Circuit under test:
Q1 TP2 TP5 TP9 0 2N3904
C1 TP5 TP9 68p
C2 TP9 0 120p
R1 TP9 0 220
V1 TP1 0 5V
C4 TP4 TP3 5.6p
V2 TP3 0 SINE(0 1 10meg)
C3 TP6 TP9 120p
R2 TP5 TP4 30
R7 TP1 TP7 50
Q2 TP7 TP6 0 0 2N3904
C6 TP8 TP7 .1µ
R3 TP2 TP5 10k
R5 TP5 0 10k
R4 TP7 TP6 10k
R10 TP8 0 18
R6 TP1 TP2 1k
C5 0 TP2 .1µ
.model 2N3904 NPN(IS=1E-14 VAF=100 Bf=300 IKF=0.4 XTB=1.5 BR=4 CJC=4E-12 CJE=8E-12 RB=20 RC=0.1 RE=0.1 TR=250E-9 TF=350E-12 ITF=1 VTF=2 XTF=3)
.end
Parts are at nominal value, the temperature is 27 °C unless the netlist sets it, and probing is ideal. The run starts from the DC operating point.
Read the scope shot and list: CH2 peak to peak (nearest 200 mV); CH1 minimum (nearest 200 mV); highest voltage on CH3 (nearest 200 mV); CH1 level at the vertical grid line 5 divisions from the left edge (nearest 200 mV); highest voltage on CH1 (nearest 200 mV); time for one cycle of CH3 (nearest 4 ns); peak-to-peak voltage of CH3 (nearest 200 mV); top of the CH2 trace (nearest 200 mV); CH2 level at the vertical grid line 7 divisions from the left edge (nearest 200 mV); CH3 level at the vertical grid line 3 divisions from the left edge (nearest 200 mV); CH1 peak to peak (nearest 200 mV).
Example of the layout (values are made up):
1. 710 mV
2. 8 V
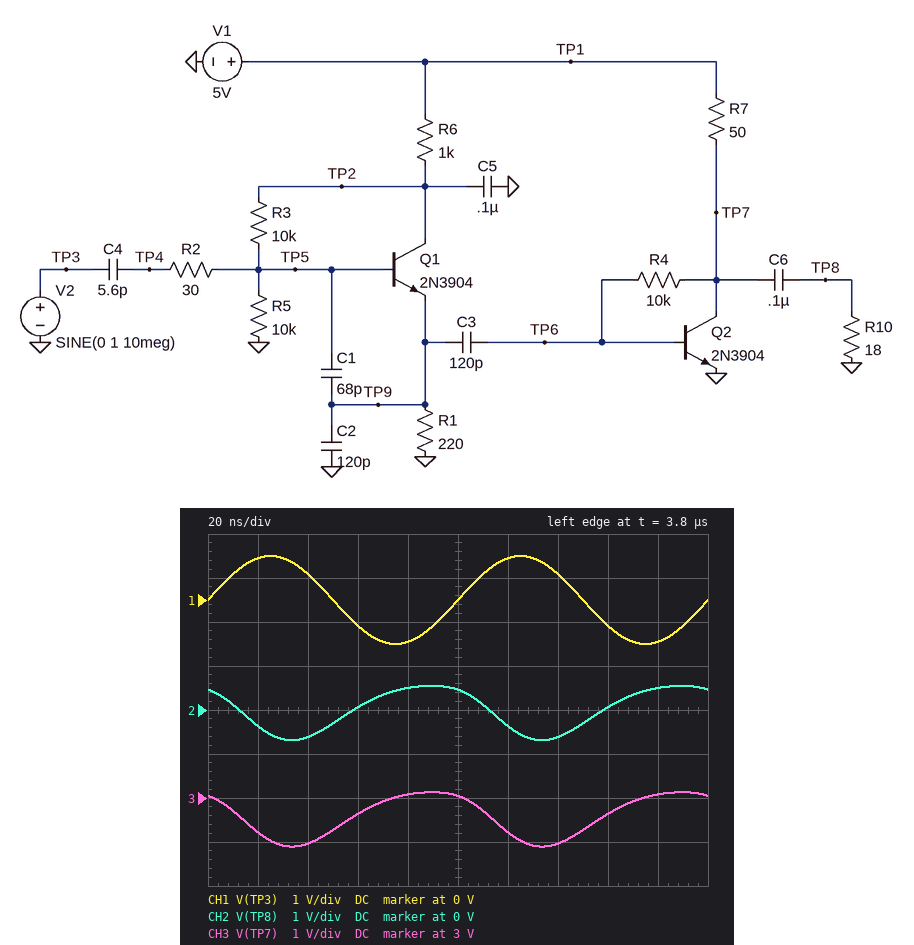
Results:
1. 1.2 V
2. -1.0 V
3. 3.2 V
4. 0 V
5. 1.0 V
6. 100 ns
7. 1.2 V
8. 600 mV
9. -600 mV
10. 2.6 V
11. 2.0 V
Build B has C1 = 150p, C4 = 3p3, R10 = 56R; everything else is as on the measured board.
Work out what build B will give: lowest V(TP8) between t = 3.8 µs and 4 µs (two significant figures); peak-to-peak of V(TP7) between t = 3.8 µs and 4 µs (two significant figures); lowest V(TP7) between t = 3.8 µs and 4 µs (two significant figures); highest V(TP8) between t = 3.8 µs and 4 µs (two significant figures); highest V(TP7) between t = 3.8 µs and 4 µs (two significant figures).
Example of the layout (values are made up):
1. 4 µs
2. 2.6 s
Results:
1. -570 mV
2. 1.1 V
3. 2.0 V
4. 520 mV
5. 3.1 V
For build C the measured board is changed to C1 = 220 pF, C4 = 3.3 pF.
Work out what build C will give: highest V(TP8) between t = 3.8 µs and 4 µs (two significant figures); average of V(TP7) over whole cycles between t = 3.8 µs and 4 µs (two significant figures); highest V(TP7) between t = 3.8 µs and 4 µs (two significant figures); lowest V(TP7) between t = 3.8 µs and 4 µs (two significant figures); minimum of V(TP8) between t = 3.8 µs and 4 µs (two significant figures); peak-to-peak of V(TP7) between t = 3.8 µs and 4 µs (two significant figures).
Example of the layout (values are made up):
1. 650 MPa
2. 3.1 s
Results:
1. 220 mV
2. 2.6 V
3. 2.8 V
4. 2.3 V
5. -240 mV
6. 450 mV
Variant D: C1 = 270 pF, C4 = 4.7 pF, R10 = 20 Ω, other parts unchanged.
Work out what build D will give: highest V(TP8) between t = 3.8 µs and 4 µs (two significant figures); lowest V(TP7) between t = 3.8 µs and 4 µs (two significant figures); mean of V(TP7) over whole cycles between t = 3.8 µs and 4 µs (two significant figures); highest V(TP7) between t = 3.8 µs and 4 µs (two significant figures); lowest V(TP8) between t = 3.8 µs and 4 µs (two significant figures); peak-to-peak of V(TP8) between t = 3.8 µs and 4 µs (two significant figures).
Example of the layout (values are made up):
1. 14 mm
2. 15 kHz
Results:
1. 270 mV
2. 2.3 V
3. 2.6 V
4. 2.8 V
5. -300 mV
6. 570 mV
